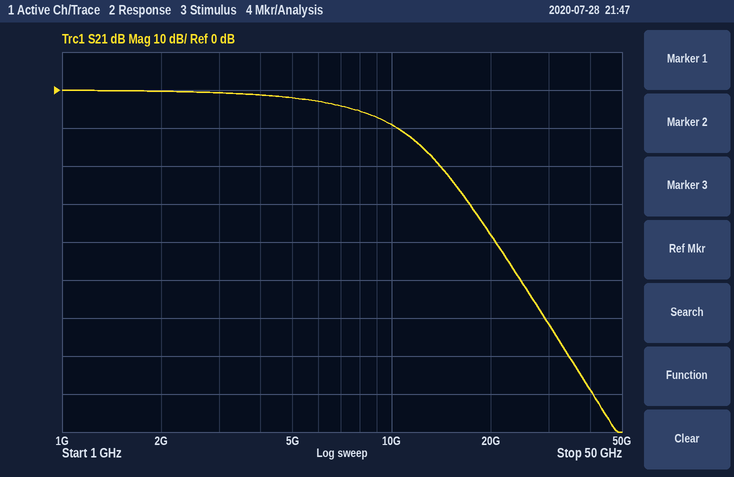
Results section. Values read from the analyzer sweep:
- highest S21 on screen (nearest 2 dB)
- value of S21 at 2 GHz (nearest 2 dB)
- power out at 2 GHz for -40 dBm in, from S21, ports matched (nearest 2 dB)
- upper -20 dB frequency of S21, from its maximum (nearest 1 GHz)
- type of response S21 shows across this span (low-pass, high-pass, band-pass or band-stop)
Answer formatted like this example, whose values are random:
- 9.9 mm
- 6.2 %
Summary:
- 0 dB
- 0 dB
- -40 dBm
- 14 GHz
- low-pass
